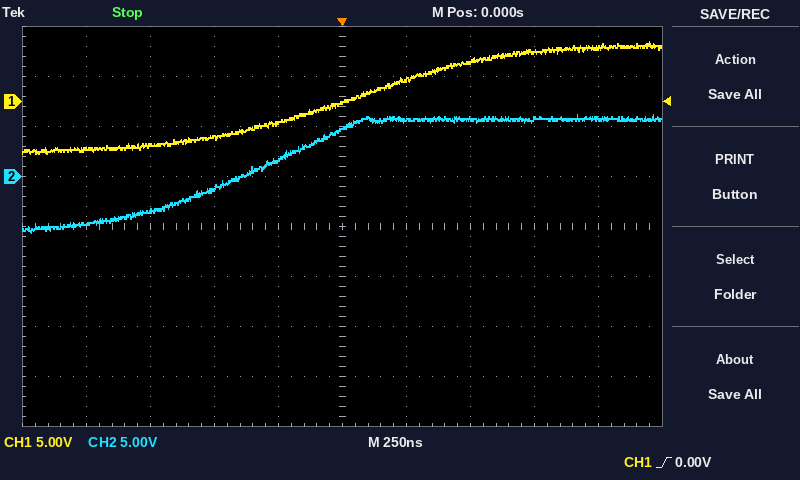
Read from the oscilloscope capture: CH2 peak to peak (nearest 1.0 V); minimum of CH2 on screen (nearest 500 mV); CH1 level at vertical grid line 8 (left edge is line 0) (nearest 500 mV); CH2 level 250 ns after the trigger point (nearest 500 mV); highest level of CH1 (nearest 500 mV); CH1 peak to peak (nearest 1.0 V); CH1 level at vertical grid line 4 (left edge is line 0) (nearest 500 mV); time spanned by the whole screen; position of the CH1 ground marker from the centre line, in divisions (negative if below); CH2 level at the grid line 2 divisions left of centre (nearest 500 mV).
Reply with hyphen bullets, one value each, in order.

- 12.0 V
- -5.5 V
- 5.0 V
- 5.5 V
- 6.0 V
- 11.0 V
- -2.0 V
- 2.5 µs
- +2.5 div
- -1.0 V
